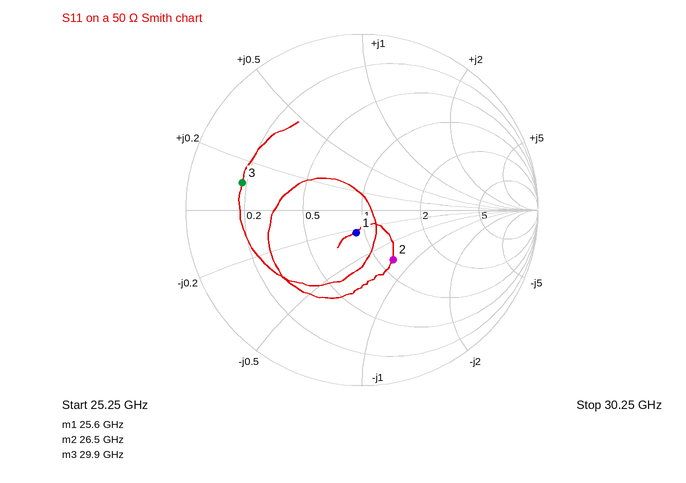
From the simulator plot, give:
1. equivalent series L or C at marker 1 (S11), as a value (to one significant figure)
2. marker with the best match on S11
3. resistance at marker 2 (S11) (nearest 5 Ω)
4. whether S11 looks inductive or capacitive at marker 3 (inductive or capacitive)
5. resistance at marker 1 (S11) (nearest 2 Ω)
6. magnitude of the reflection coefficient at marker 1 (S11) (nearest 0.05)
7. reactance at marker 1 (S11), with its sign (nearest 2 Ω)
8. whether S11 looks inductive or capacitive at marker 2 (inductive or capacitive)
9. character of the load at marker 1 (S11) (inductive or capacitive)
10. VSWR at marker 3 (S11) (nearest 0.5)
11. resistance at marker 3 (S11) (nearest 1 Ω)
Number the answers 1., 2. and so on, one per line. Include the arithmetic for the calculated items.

1. C = 1/(2π × 25.6 GHz × 12 Ω) ≈ 518 fF, so 500 fF to one significant figure
2. marker 1
3. 60 Ω
4. inductive
5. 46 Ω
6. 0.15
7. -12 Ω
8. capacitive
9. capacitive
10. 5.5
11. 9 Ω
